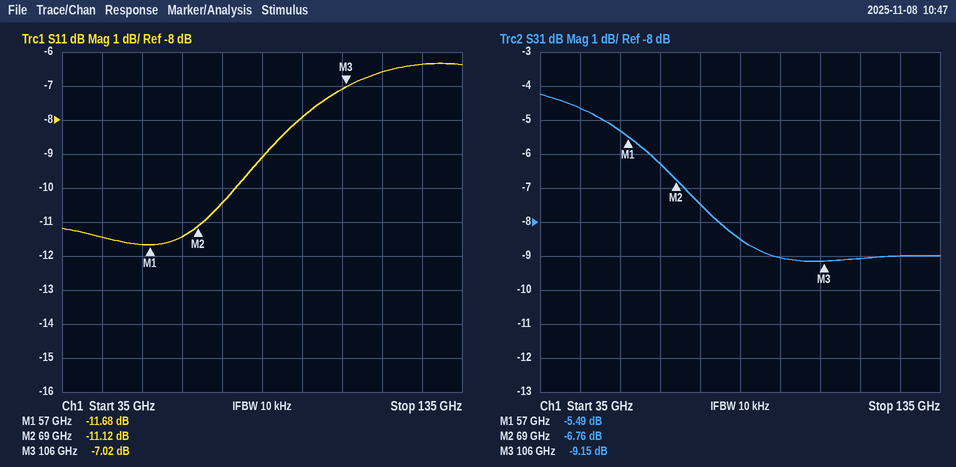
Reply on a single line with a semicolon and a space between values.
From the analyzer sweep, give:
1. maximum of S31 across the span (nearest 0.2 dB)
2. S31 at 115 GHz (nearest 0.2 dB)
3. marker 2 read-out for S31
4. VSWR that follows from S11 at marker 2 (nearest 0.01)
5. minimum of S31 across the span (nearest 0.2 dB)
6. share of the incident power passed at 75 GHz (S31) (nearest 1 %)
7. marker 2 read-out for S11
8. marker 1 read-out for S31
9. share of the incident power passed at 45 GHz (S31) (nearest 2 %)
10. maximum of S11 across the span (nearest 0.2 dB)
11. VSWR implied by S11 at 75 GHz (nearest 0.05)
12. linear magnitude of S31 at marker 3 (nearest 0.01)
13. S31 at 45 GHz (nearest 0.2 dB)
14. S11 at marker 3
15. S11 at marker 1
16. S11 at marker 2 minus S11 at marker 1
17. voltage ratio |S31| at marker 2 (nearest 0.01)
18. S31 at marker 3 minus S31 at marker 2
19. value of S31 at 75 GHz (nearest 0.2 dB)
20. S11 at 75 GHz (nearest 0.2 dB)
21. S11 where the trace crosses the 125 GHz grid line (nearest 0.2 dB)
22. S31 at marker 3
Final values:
-4.2 dB; -9.0 dB; -6.76 dB; 1.77; -9.2 dB; 18 %; -11.12 dB; -5.49 dB; 34 %; -6.4 dB; 1.85; 0.35; -4.6 dB; -7.02 dB; -11.68 dB; 0.56 dB; 0.46; -2.39 dB; -7.4 dB; -10.4 dB; -6.4 dB; -9.15 dB
